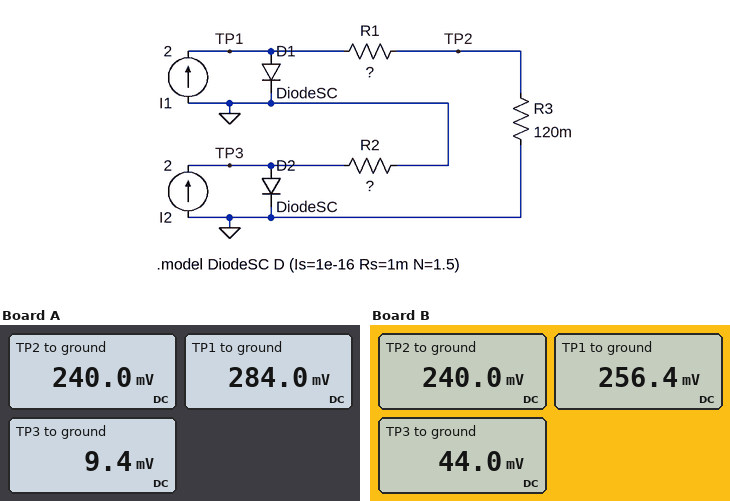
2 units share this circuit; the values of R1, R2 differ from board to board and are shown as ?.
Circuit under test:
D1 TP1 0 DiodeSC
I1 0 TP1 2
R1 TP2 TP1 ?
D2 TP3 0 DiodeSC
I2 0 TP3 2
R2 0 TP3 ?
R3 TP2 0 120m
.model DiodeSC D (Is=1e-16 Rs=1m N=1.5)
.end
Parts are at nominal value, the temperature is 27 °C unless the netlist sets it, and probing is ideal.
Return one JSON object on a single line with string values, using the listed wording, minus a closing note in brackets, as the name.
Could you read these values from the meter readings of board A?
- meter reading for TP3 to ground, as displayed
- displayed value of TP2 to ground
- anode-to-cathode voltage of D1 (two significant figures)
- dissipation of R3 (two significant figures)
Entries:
{"meter reading for TP3 to ground, as displayed": "9.4 mV", "displayed value of TP2 to ground": "240.0 mV", "anode-to-cathode voltage of D1": "280 mV", "dissipation of R3": "480 mW"}
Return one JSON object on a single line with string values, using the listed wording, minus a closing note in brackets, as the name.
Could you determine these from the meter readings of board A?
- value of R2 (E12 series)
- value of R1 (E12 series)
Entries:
{"value of R2": "4.7 mΩ", "value of R1": "0.022 Ω"}
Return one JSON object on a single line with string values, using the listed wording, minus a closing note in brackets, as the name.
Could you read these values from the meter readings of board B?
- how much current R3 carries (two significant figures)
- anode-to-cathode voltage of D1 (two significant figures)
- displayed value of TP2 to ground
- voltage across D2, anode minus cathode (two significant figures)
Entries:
{"how much current R3 carries": "2.0 A", "anode-to-cathode voltage of D1": "260 mV", "displayed value of TP2 to ground": "240.0 mV", "voltage across D2, anode minus cathode": "44 mV"}
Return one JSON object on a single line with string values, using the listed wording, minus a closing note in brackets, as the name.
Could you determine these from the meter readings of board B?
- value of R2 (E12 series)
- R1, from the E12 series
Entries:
{"value of R2": "0.022 Ω", "R1, from the E12 series": "8.2 mΩ"}
